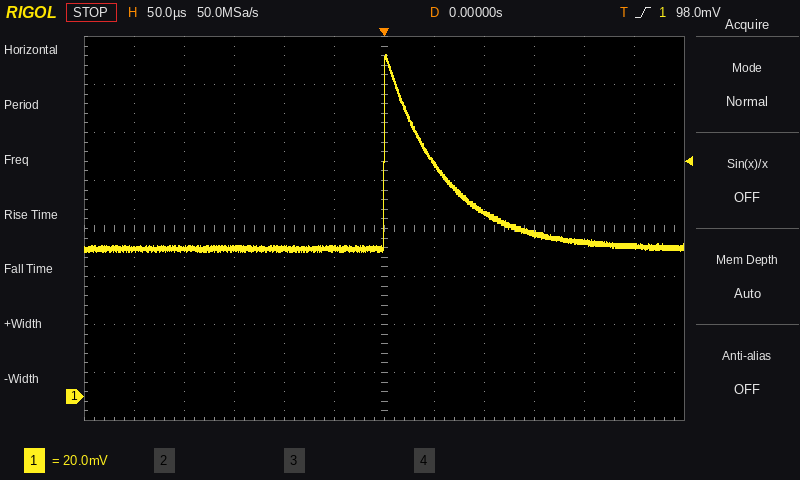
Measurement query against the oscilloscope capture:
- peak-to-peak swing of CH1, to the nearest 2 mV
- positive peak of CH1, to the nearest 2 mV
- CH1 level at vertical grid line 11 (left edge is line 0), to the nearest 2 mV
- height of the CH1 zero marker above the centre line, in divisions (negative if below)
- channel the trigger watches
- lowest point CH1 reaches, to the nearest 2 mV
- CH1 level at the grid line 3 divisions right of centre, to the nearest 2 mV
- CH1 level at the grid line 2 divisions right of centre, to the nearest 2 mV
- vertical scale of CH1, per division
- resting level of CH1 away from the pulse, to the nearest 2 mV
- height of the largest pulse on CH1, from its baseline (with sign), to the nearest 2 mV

82 mV
142 mV
62 mV
-3.5 div
CH1
60 mV
68 mV
76 mV
20 mV
62 mV
+80 mV
